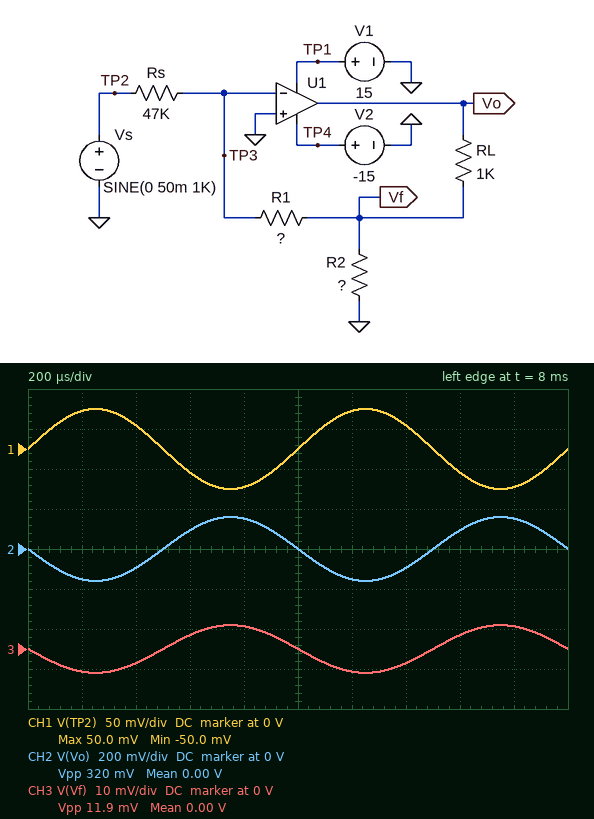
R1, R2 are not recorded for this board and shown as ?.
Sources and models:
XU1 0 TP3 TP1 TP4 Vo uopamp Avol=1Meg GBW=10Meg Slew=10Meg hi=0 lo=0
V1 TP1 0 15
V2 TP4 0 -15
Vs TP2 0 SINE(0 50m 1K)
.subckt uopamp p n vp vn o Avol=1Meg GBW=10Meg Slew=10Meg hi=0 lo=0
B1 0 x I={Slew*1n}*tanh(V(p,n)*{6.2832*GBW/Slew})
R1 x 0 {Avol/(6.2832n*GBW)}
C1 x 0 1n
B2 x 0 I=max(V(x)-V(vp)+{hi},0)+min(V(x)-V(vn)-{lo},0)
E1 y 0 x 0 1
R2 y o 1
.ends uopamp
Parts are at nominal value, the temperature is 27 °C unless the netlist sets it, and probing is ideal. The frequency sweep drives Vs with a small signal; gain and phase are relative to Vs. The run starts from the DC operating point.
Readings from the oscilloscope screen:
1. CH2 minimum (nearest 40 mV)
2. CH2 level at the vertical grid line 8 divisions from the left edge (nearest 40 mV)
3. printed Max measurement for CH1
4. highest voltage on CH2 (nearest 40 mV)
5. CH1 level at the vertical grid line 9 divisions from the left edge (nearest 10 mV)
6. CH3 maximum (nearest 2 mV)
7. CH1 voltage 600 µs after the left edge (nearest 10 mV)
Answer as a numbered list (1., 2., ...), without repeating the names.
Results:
1. -160 mV
2. 80 mV
3. 50.0 mV
4. 160 mV
5. -50 mV
6. 6 mV
7. -30 mV
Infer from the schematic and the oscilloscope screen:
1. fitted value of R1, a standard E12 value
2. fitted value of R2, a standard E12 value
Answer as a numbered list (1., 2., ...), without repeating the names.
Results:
1. 5.6 kΩ
2. 39 Ω
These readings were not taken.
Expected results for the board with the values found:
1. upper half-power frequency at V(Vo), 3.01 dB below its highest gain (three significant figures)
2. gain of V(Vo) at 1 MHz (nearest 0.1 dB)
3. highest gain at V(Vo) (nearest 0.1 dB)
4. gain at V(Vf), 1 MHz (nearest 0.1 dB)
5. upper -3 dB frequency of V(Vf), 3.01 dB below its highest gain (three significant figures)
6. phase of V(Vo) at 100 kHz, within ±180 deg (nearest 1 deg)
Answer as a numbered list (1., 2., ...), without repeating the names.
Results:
1. 335 kHz
2. 0.1 dB
3. 10.1 dB
4. -28.4 dB
5. 335 kHz
6. 163 deg
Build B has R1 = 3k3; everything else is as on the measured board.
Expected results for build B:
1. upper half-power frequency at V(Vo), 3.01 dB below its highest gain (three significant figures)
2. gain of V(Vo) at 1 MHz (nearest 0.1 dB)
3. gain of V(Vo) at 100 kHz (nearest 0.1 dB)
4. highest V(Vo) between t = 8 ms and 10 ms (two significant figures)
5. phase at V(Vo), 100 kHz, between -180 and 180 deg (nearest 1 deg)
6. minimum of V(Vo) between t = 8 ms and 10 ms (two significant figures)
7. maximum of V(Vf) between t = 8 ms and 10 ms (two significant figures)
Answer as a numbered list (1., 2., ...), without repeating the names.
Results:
1. 350 kHz
2. -4.1 dB
3. 5.2 dB
4. 95 mV
5. 164 deg
6. -95 mV
7. 3.5 mV
